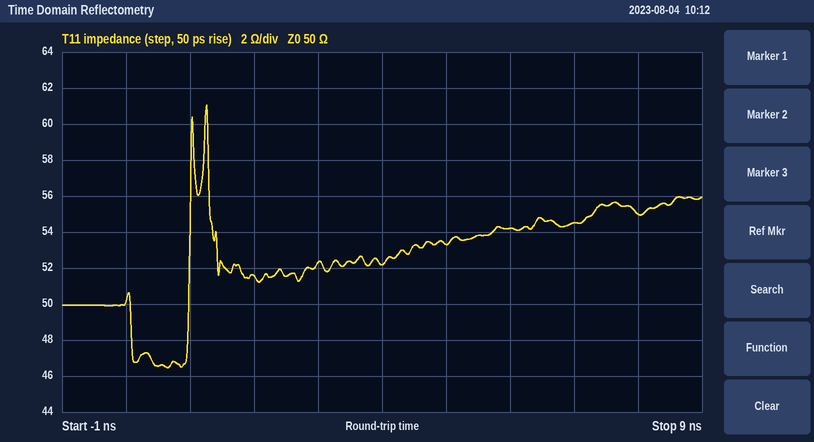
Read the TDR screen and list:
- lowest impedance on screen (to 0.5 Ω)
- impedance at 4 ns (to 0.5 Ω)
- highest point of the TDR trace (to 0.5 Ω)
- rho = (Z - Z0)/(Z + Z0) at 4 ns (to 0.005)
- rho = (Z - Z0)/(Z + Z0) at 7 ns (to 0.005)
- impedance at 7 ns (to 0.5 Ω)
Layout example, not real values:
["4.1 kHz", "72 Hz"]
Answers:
["46.5 Ω", "52.0 Ω", "61.0 Ω", "+0.020", "+0.045", "54.5 Ω"]
